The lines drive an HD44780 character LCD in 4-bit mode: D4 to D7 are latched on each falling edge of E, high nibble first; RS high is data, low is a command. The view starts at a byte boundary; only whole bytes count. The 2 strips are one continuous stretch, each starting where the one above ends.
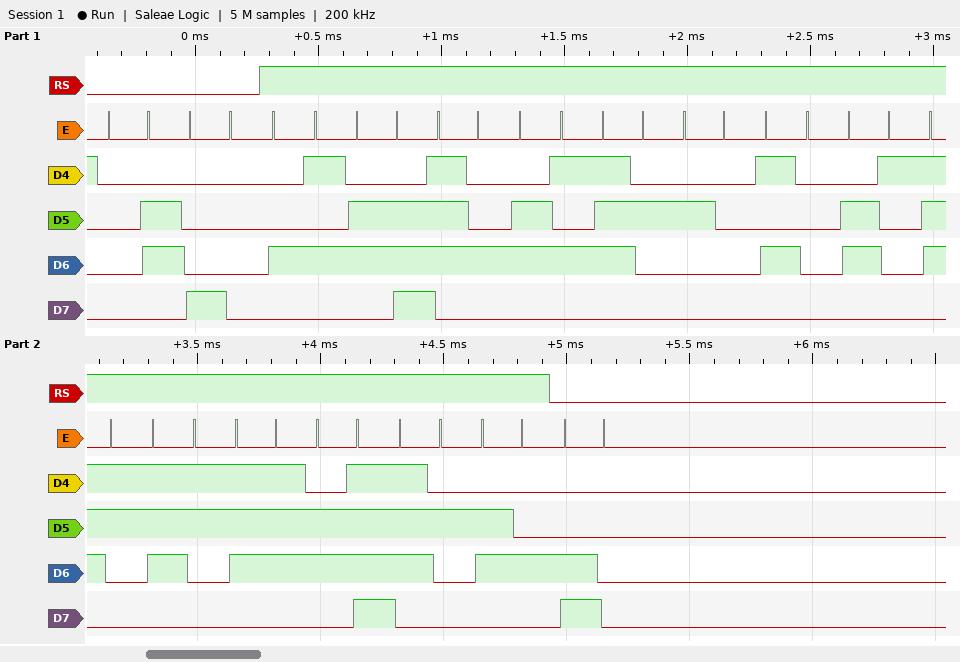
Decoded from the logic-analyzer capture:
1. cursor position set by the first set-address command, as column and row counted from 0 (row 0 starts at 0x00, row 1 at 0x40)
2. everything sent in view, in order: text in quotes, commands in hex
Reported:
column 0, row 0
0x06 0x80 "Enter Password" 0xC0
